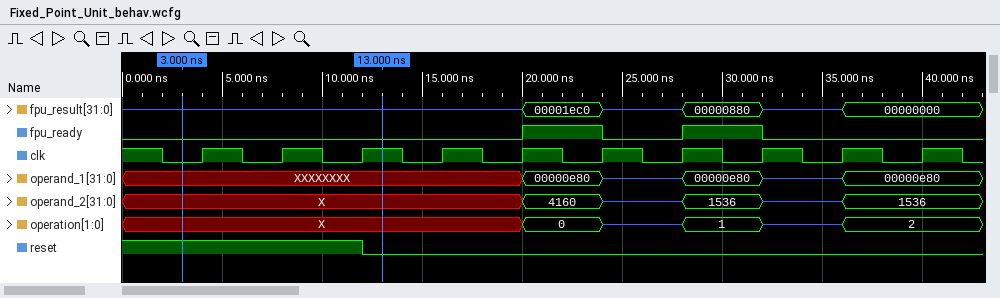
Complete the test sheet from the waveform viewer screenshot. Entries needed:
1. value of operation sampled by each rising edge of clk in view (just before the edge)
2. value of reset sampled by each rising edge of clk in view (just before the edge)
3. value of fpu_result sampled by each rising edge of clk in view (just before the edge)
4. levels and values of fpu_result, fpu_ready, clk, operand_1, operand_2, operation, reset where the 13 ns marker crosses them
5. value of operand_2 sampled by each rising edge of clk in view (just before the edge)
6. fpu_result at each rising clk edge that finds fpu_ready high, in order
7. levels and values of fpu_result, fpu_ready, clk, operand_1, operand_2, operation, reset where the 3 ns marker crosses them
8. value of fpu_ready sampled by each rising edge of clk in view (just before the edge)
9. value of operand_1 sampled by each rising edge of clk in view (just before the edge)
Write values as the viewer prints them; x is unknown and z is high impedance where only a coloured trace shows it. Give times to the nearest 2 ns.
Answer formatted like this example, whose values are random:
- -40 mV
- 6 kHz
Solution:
- X, X, X, X, X, 0, z, 1, z, 2
- 1 1 1 0 0 0 0 0 0 0
- z, z, z, z, z, 00001ec0, z, 00000880, z, 00000000
- fpu_result=z, fpu_ready=0, clk=1, operand_1=XXXXXXXX, operand_2=X, operation=X, reset=0
- X, X, X, X, X, 4160, z, 1536, z, 1536
- 00001ec0, 00000880
- fpu_result=z, fpu_ready=0, clk=0, operand_1=XXXXXXXX, operand_2=X, operation=X, reset=1
- 0 0 0 0 0 1 0 1 0 0
- XXXXXXXX, XXXXXXXX, XXXXXXXX, XXXXXXXX, XXXXXXXX, 00000e80, z, 00000e80, z, 00000e80
